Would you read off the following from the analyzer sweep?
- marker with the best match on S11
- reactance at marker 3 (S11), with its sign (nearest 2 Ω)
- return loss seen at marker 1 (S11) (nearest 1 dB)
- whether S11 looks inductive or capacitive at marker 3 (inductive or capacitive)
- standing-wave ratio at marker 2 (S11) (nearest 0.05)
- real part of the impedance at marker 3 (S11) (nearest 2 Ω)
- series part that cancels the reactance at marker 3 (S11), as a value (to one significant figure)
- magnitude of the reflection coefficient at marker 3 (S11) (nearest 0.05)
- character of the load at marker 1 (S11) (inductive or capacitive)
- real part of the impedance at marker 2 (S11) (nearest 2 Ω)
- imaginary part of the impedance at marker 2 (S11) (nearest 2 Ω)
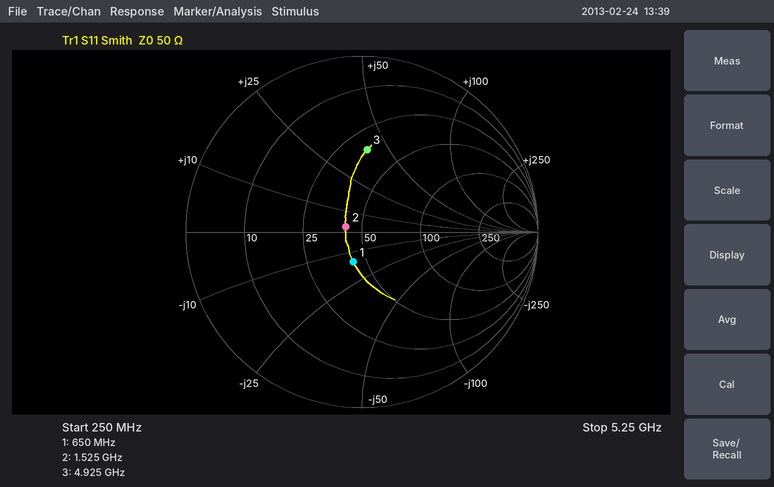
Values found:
marker 2
+40 Ω
15 dB
inductive
1.20
34 Ω
800 fF
0.45
capacitive
42 Ω
+2 Ω
